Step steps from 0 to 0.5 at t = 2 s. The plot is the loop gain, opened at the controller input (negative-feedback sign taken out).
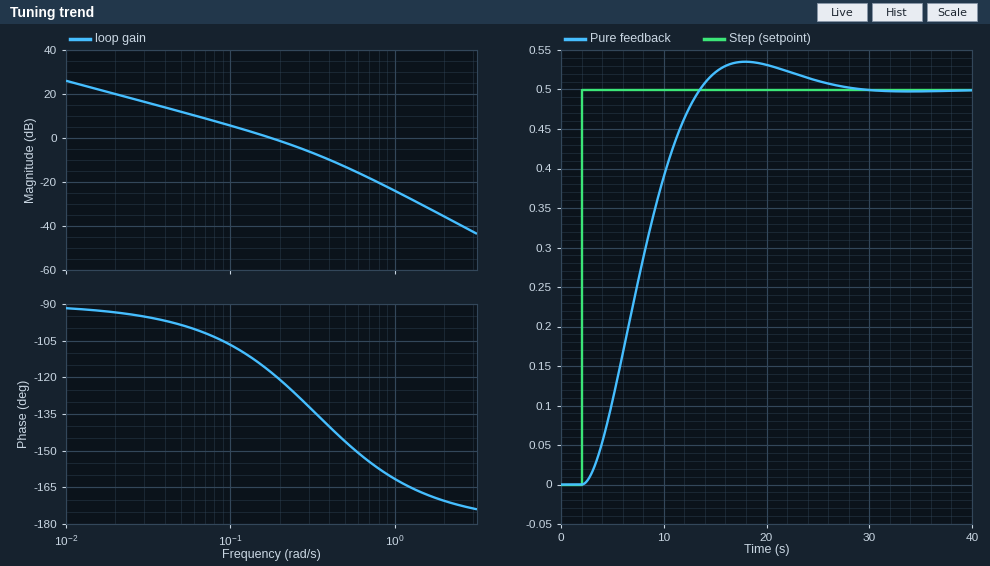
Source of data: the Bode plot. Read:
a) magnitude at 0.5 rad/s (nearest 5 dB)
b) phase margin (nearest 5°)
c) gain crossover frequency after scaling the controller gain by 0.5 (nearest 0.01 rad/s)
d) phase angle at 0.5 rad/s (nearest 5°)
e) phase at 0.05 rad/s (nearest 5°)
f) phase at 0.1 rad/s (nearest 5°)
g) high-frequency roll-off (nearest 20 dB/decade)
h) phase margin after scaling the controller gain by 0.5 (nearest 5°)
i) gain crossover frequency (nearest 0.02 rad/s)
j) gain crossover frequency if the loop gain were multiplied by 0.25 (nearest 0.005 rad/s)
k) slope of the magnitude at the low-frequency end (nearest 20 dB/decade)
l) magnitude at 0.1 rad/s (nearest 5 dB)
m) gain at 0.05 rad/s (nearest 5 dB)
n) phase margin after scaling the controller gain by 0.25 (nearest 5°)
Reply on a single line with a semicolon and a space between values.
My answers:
-15 dB; 60°; 0.10 rad/s; -145°; -100°; -105°; -40 dB/decade; 75°; 0.18 rad/s; 0.050 rad/s; -20 dB/decade; 5 dB; 10 dB; 80°
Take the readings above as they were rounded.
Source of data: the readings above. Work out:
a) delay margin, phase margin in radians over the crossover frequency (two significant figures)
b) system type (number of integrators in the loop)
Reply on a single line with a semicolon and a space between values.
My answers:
5.8 s; 1
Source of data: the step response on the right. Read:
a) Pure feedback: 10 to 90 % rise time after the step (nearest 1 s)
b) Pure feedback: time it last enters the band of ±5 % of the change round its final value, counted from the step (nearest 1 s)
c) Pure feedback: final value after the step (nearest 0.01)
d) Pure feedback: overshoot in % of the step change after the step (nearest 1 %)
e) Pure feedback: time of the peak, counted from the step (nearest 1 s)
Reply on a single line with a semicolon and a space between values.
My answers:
8 s; 20 s; 0.50; 7 %; 16 s
